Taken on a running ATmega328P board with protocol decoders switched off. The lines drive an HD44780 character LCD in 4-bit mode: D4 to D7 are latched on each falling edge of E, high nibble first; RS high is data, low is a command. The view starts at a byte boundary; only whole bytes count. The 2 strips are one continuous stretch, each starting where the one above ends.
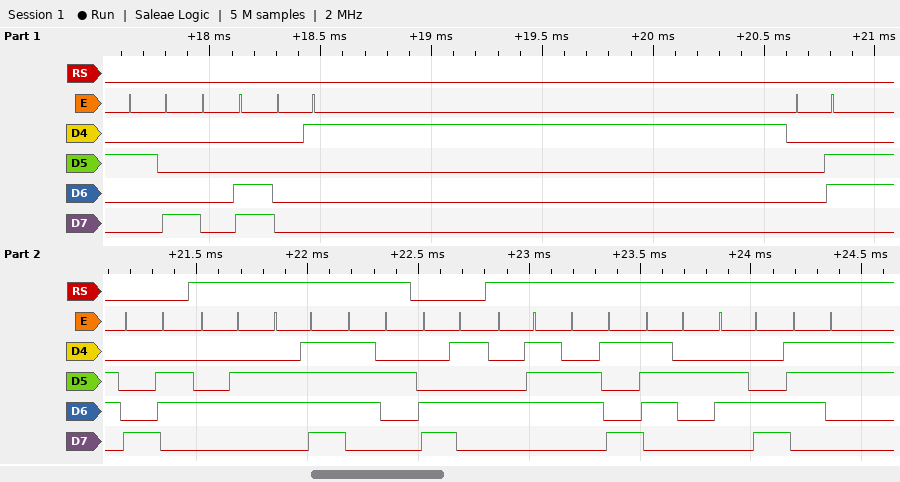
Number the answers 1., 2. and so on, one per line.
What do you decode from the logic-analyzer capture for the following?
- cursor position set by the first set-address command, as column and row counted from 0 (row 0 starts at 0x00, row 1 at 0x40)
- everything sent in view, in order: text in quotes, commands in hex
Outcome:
1. column 6, row 0
2. 0x28 0x0C 0x01 0x06 0x86 "For" 0xC5 "Girls"
